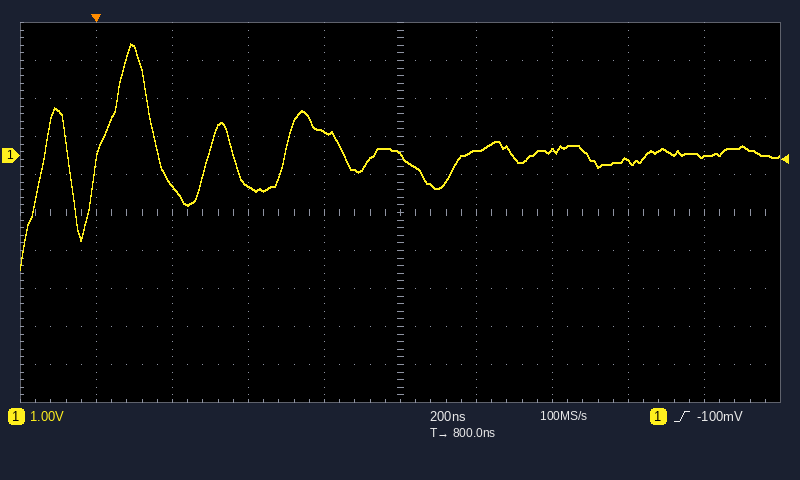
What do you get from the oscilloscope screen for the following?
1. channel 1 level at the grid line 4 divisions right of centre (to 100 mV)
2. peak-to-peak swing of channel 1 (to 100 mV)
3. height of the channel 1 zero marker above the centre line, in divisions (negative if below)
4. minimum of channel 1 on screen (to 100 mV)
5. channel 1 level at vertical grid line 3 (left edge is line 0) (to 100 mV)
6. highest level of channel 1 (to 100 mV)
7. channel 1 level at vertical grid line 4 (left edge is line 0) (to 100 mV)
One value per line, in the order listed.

0.0 V
5.9 V
+1.5 div
-3.0 V
-800 mV
2.9 V
600 mV
